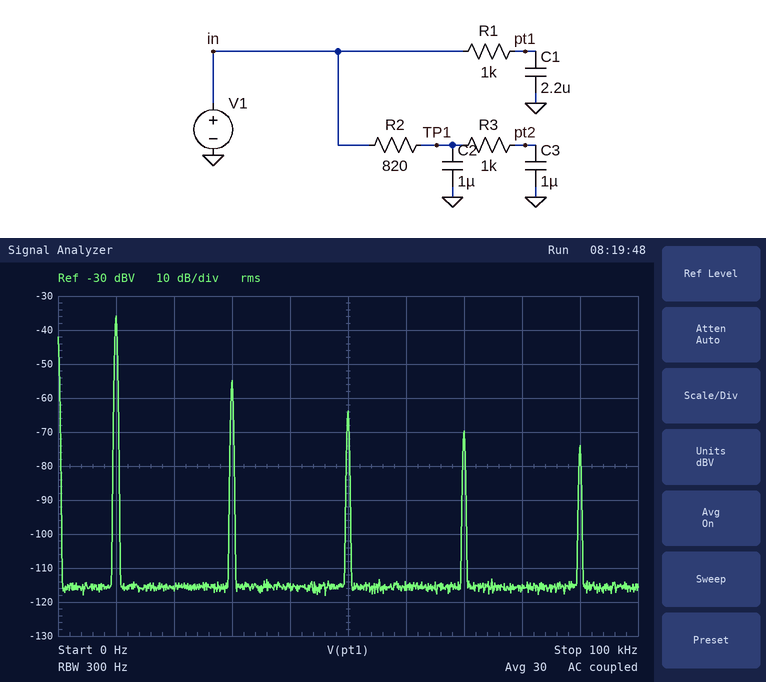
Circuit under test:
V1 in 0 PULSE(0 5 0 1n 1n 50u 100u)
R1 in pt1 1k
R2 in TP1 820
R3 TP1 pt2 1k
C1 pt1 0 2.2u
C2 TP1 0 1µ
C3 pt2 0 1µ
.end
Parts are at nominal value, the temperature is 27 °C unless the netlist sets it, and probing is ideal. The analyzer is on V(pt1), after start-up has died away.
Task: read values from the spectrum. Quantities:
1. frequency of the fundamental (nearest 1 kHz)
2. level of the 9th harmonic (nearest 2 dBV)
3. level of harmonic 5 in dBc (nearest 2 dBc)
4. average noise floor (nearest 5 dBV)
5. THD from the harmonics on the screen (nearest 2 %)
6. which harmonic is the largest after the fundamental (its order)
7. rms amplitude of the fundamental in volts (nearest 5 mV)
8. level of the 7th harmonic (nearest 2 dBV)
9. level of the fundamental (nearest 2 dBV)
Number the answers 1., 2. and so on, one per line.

1. 10 kHz
2. -74 dBV
3. -28 dBc
4. -115 dBV
5. 12 %
6. 3
7. 15 mV
8. -70 dBV
9. -36 dBV
